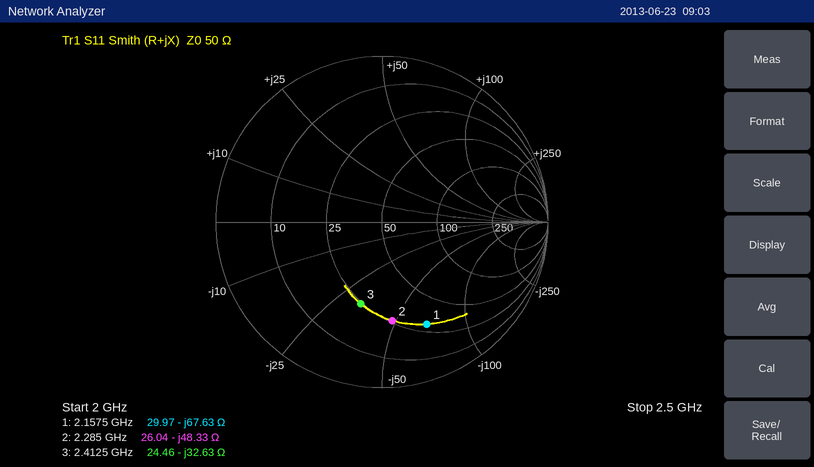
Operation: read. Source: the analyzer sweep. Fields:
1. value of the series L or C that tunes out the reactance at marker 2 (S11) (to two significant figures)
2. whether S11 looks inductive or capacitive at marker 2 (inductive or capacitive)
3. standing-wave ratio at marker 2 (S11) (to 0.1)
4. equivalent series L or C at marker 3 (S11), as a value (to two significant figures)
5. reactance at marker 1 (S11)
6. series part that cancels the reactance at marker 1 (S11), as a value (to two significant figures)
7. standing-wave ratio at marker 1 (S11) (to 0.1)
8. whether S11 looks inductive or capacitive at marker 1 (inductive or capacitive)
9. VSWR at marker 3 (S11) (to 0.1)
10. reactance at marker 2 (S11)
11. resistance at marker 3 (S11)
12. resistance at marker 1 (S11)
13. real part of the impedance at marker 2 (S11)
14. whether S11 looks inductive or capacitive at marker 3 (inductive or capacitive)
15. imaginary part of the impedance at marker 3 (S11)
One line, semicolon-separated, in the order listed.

3.4 nH; capacitive; 4.0; 2.0 pF; -67.63 Ω; 5.0 nH; 5.1; capacitive; 3.1; -48.33 Ω; 24.46 Ω; 29.97 Ω; 26.04 Ω; capacitive; -32.63 Ω
